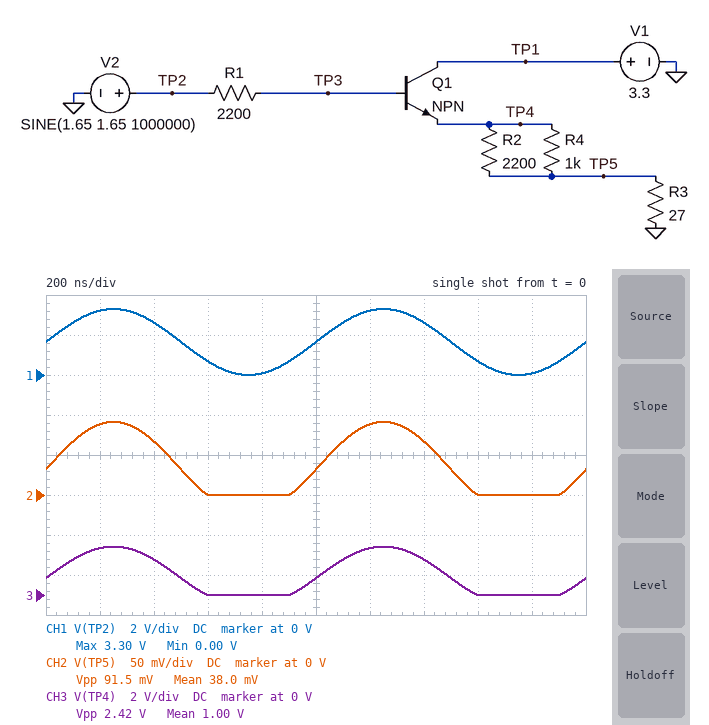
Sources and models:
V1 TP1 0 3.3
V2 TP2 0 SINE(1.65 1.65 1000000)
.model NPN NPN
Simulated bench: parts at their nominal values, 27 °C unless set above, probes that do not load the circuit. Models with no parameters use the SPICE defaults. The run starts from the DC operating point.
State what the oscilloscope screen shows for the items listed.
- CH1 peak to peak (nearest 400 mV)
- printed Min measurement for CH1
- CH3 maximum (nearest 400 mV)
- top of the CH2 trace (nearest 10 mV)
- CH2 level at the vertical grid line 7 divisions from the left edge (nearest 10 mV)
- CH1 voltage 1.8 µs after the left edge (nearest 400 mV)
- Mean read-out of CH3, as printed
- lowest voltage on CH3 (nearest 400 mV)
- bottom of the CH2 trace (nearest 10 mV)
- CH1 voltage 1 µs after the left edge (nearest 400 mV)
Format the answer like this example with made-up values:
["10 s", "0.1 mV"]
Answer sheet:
["3.2 V", "0.00 V", "2.4 V", "90 mV", "70 mV", "0 V", "1.00 V", "0 V", "0 V", "1.6 V"]
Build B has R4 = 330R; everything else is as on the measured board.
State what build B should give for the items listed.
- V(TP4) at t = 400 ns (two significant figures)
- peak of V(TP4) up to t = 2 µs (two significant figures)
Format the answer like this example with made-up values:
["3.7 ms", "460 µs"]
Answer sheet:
["1.7 V", "2.3 V"]
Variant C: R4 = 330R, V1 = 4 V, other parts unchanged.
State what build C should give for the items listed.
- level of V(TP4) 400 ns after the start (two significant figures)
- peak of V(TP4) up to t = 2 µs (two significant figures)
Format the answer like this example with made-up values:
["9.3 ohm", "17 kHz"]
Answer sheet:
["1.7 V", "2.3 V"]
